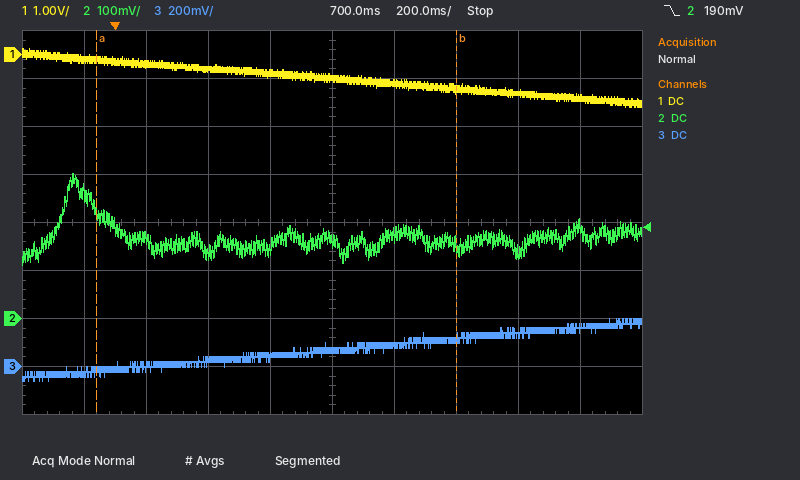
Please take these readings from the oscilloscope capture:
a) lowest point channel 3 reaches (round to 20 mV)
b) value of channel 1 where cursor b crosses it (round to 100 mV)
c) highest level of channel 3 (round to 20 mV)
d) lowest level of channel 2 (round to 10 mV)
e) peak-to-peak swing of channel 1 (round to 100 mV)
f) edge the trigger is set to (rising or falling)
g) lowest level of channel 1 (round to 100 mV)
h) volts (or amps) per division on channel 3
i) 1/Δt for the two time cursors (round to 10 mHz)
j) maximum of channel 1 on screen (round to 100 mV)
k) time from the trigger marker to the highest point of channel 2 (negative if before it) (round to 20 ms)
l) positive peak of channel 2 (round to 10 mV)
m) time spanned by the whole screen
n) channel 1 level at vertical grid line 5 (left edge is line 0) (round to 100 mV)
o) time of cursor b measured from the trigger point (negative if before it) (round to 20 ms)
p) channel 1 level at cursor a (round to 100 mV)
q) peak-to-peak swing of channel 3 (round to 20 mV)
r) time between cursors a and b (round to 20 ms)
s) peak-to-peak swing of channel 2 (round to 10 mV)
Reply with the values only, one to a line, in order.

-60 mV
-700 mV
200 mV
110 mV
1.2 V
falling
-1.1 V
200 mV
860 mHz
100 mV
-140 ms
300 mV
2 s
-500 mV
+1.10 s
-100 mV
260 mV
1.16 s
190 mV
